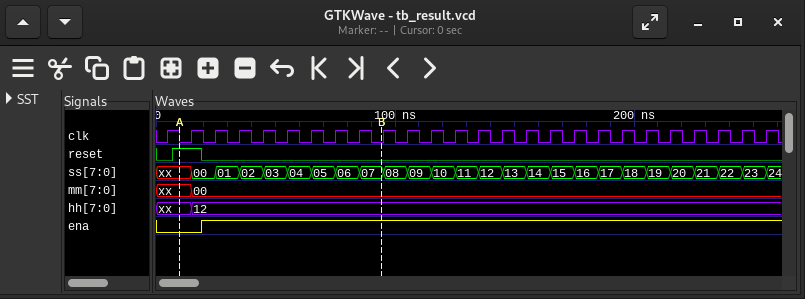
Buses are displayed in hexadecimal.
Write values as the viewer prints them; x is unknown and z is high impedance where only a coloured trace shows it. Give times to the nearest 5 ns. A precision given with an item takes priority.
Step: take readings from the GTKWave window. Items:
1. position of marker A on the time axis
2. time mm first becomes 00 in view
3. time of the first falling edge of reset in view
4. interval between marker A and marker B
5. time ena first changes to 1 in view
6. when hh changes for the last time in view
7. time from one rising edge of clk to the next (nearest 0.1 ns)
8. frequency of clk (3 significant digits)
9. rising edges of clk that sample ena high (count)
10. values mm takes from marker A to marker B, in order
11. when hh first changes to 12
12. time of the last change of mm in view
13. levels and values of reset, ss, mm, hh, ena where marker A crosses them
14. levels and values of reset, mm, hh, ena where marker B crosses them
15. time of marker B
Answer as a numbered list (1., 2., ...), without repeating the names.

1. 10 ns
2. 15 ns
3. 20 ns
4. 85 ns
5. 20 ns
6. 15 ns
7. 10 ns
8. 100 MHz
9. 24
10. xx, 00
11. 15 ns
12. 15 ns
13. reset=1, ss=xx, mm=xx, hh=xx, ena=0
14. reset=0, mm=00, hh=12, ena=1
15. 95 ns
